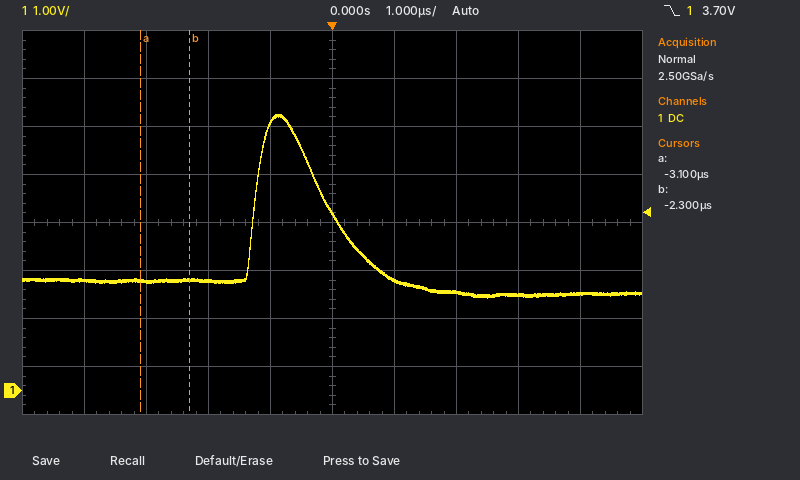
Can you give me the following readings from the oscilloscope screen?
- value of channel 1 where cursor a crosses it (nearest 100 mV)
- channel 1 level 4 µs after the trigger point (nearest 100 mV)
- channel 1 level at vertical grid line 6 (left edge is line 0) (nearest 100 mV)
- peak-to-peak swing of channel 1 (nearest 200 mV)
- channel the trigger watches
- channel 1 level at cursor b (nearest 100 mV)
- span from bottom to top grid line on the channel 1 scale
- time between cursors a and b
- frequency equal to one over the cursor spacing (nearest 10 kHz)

2.3 V
2.0 V
2.3 V
3.8 V
channel 1
2.3 V
8 V
800 ns
1.25 MHz
